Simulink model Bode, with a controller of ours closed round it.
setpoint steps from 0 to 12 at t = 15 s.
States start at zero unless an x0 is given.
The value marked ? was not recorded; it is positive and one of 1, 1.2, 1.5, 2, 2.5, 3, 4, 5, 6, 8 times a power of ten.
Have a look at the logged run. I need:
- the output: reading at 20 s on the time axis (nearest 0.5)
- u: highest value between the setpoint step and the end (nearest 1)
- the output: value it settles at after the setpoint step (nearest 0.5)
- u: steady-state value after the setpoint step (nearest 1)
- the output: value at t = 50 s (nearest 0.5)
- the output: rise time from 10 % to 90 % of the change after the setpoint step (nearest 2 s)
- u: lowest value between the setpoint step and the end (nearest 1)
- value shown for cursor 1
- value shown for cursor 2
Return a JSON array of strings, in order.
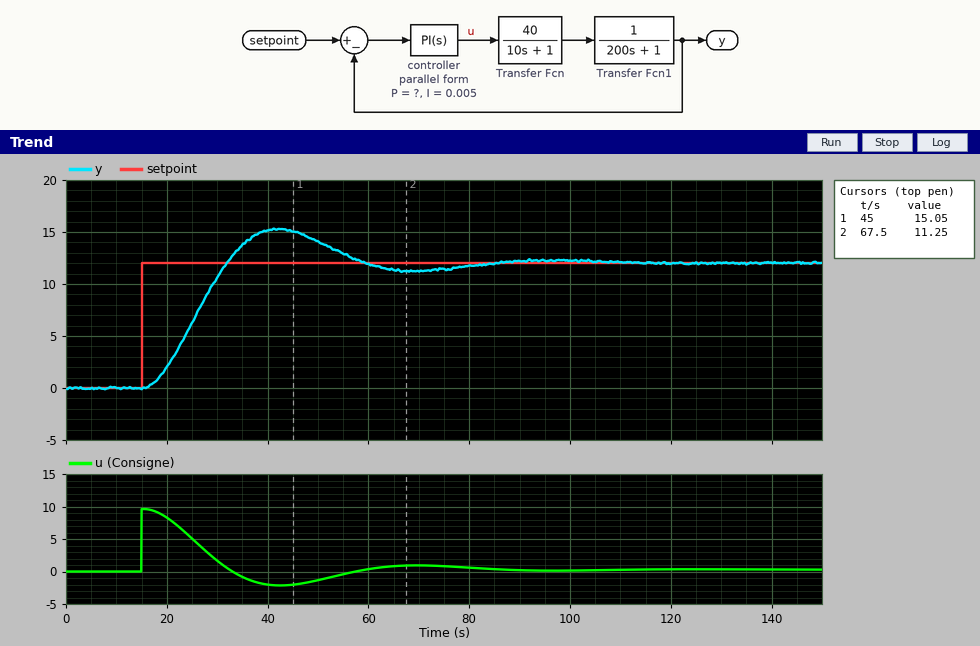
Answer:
["2.0", "10", "12.0", "0", "14.0", "12 s", "-2", "15.05", "11.25"]
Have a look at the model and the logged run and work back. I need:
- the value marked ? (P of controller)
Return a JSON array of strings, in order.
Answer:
["0.8"]
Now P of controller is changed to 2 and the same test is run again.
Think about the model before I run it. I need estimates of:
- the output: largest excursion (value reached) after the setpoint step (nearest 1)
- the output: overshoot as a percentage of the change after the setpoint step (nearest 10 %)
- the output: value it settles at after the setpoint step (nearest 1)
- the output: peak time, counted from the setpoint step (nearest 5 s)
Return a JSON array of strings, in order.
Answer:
["17", "40 %", "12", "15 s"]
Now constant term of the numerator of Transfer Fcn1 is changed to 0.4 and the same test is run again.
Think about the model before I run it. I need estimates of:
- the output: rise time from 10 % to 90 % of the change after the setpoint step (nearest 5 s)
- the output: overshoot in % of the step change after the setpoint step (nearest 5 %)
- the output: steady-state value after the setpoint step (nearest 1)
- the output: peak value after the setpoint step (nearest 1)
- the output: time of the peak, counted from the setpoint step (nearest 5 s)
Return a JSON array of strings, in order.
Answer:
["25 s", "10 %", "12", "13", "50 s"]
